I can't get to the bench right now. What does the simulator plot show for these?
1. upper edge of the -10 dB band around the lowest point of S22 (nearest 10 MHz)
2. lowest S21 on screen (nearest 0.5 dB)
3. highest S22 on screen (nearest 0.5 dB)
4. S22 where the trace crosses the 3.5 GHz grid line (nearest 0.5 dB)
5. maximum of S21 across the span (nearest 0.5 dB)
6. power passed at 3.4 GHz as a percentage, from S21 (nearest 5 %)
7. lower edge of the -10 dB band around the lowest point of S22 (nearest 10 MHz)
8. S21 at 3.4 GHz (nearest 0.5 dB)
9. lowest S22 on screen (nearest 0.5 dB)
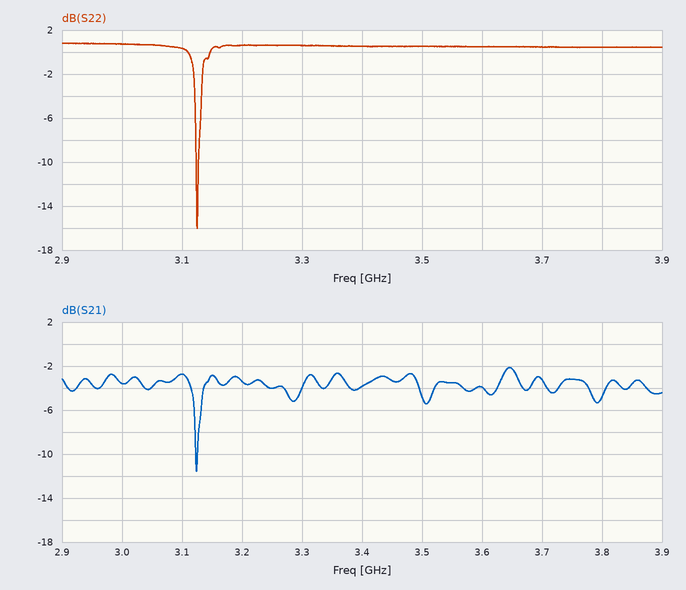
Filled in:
3.13 GHz
-11.5 dB
1.0 dB
0.5 dB
-2.0 dB
40 %
3.12 GHz
-4.0 dB
-16.0 dB
